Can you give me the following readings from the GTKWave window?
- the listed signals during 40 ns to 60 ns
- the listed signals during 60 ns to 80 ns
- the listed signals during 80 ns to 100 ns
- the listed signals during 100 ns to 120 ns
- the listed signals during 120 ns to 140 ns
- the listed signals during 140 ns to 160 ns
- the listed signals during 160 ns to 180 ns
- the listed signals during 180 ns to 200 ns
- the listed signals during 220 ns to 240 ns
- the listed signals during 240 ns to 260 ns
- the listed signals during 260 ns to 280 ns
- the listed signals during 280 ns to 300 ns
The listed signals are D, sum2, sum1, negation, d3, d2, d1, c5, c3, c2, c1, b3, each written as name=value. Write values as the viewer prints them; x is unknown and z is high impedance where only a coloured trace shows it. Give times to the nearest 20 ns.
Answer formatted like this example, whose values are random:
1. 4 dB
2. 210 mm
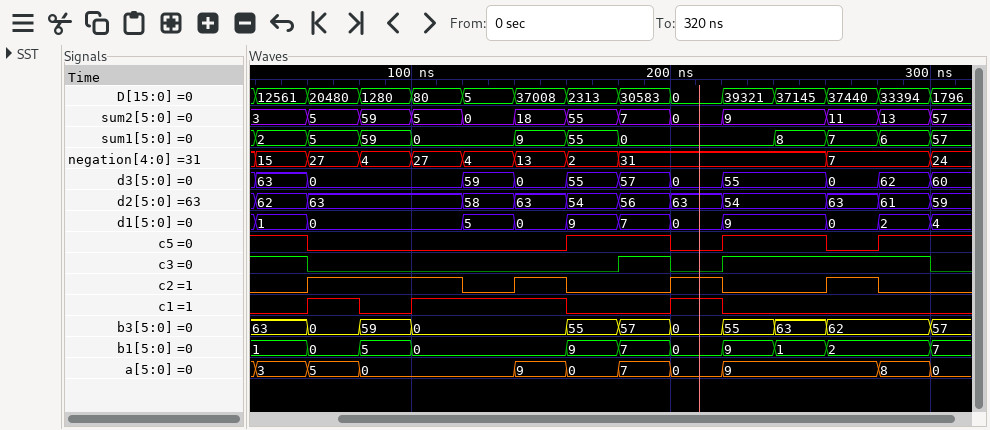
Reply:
1. D=12561, sum2=3, sum1=2, negation=15, d3=63, d2=62, d1=1, c5=1, c3=1, c2=0, c1=0, b3=63
2. D=20480, sum2=5, sum1=5, negation=27, d3=0, d2=63, d1=0, c5=0, c3=0, c2=1, c1=1, b3=0
3. D=1280, sum2=59, sum1=59, negation=4, d3=0, d2=63, d1=0, c5=0, c3=0, c2=1, c1=0, b3=59
4. D=80, sum2=5, sum1=0, negation=27, d3=0, d2=63, d1=0, c5=0, c3=0, c2=1, c1=1, b3=0
5. D=5, sum2=0, sum1=0, negation=4, d3=59, d2=58, d1=5, c5=0, c3=0, c2=0, c1=1, b3=0
6. D=37008, sum2=18, sum1=9, negation=13, d3=0, d2=63, d1=0, c5=0, c3=0, c2=1, c1=1, b3=0
7. D=2313, sum2=55, sum1=55, negation=2, d3=55, d2=54, d1=9, c5=1, c3=0, c2=0, c1=0, b3=55
8. D=30583, sum2=7, sum1=0, negation=31, d3=57, d2=56, d1=7, c5=1, c3=1, c2=0, c1=0, b3=57
9. D=39321, sum2=9, sum1=0, negation=31, d3=55, d2=54, d1=9, c5=1, c3=1, c2=0, c1=0, b3=55
10. D=37145, sum2=9, sum1=8, negation=31, d3=55, d2=54, d1=9, c5=1, c3=1, c2=0, c1=0, b3=63
11. D=37440, sum2=11, sum1=7, negation=7, d3=0, d2=63, d1=0, c5=0, c3=1, c2=1, c1=0, b3=62
12. D=33394, sum2=13, sum1=6, negation=7, d3=62, d2=61, d1=2, c5=1, c3=1, c2=0, c1=0, b3=62
